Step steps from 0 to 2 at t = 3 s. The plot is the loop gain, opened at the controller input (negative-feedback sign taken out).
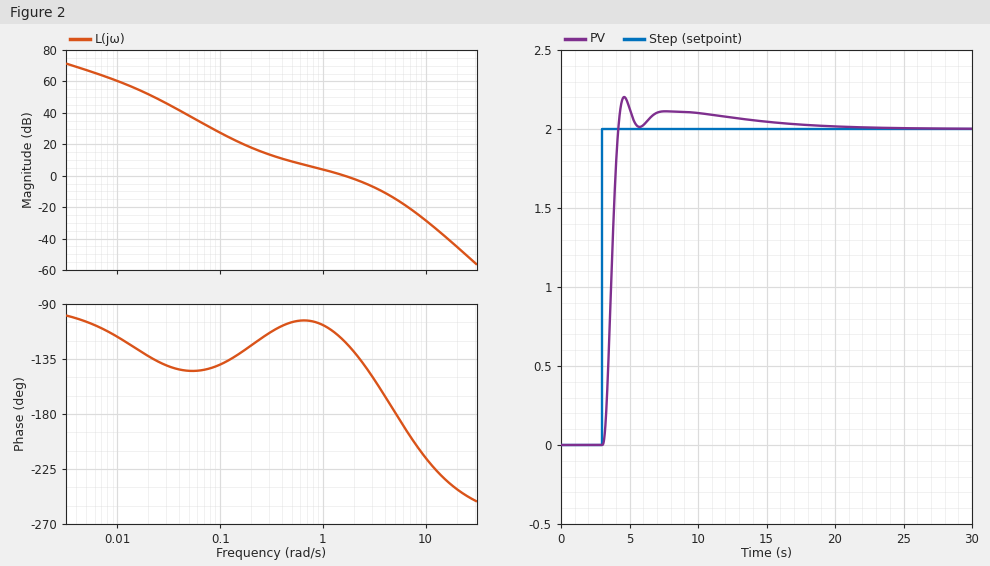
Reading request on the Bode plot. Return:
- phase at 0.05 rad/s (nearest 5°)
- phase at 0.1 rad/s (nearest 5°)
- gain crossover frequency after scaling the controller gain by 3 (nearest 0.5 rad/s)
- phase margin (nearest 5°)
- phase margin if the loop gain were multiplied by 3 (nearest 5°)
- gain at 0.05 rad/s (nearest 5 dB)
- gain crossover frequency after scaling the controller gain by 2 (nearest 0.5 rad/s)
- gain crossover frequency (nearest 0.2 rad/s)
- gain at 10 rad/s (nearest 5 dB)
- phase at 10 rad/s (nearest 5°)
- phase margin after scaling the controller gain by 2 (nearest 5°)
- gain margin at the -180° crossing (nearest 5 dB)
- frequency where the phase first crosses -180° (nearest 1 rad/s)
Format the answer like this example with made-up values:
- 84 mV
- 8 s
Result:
- -145°
- -140°
- 3.5 rad/s
- 60°
- 20°
- 40 dB
- 3.0 rad/s
- 1.6 rad/s
- -30 dB
- -215°
- 35°
- 15 dB
- 5 rad/s
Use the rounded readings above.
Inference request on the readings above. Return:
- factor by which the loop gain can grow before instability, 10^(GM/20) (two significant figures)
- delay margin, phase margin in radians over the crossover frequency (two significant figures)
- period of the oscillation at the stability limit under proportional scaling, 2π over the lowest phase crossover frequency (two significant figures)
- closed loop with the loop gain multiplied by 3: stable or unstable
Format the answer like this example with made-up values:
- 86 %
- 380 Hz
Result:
- 5.6
- 0.65 s
- 1.3 s
- stable
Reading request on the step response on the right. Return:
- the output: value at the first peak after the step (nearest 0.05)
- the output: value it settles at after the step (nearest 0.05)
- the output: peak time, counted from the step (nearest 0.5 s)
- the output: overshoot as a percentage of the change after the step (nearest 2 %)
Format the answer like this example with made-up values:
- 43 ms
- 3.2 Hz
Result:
- 2.20
- 2.00
- 1.5 s
- 10 %
